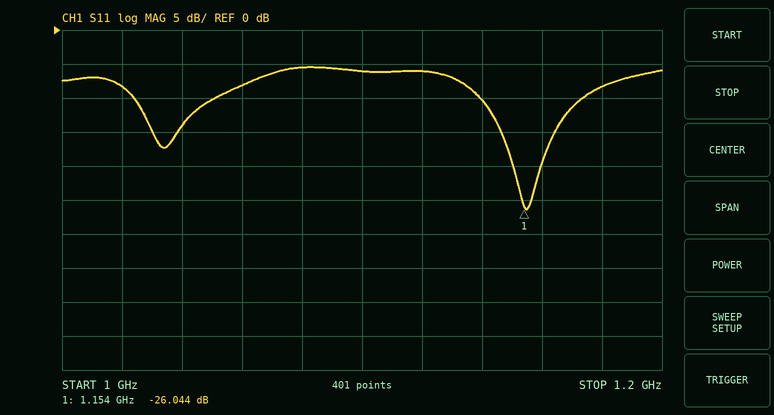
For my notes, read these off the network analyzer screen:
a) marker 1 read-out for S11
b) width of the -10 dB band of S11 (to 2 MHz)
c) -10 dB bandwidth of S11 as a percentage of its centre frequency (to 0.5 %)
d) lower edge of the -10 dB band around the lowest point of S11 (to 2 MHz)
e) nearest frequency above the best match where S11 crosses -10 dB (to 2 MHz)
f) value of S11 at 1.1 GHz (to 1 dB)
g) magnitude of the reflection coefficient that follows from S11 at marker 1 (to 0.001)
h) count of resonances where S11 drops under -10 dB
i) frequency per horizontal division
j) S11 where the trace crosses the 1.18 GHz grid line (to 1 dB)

-26.044 dB
34 MHz
3.0 %
1.140 GHz
1.174 GHz
-6 dB
0.050
2
20 MHz
-8 dB
